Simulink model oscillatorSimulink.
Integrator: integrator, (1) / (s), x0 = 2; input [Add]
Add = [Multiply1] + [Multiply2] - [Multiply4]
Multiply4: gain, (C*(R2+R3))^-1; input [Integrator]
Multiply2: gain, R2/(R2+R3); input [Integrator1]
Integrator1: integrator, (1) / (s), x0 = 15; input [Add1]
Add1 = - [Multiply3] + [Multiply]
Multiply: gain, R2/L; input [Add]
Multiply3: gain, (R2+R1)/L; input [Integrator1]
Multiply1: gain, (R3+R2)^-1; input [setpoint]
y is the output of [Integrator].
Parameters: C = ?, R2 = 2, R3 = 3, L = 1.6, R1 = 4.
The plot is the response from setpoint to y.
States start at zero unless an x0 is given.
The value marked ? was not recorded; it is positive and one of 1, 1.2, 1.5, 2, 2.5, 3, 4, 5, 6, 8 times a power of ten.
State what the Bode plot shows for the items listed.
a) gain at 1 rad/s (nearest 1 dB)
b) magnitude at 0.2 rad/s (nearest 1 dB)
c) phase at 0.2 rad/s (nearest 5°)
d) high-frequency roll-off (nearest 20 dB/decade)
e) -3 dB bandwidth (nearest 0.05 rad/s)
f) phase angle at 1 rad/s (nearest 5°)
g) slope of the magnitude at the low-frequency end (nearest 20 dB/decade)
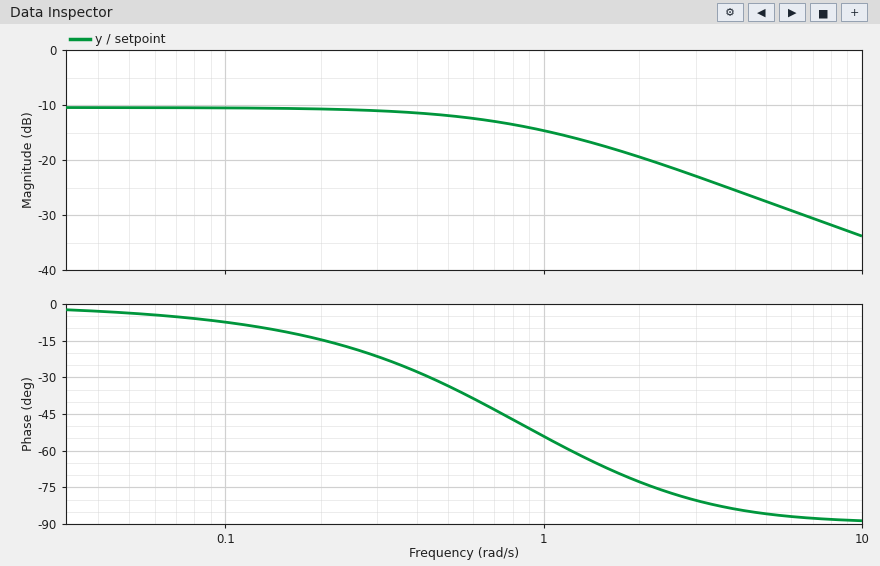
-15 dB
-11 dB
-15°
-20 dB/decade
0.80 rad/s
-55°
0 dB/decade
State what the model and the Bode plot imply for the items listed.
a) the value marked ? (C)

0.3
